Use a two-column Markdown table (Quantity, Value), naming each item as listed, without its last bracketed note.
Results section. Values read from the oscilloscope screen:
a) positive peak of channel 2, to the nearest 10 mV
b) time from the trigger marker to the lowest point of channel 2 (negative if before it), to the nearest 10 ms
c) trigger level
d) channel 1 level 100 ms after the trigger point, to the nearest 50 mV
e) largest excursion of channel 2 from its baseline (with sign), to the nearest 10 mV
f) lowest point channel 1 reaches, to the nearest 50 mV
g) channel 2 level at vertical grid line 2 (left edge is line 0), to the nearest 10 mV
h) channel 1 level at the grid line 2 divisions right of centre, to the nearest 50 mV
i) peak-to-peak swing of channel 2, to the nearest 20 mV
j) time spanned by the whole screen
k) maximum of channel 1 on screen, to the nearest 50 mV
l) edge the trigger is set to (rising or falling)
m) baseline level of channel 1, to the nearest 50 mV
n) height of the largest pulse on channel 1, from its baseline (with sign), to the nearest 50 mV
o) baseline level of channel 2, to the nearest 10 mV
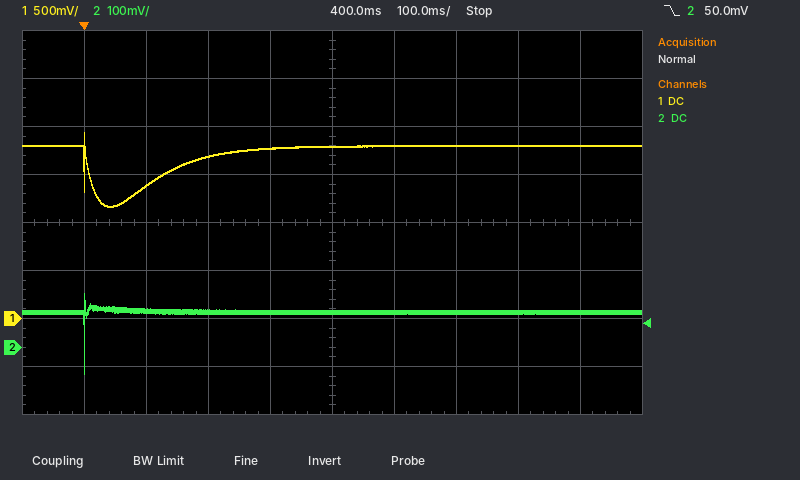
| Quantity | Value |
|---|---|
| positive peak of channel 2, to the nearest 10 mV | 110 mV |
| time from the trigger marker to the lowest point of channel 2 (negative if before it), to the nearest 10 ms | 0 ms |
| trigger level | 50.0 mV |
| channel 1 level 100 ms after the trigger point, to the nearest 50 mV | 1.40 V |
| largest excursion of channel 2 from its baseline (with sign), to the nearest 10 mV | -130 mV |
| lowest point channel 1 reaches, to the nearest 50 mV | 1.15 V |
| channel 2 level at vertical grid line 2 (left edge is line 0), to the nearest 10 mV | 80 mV |
| channel 1 level at the grid line 2 divisions right of centre, to the nearest 50 mV | 1.80 V |
| peak-to-peak swing of channel 2, to the nearest 20 mV | 160 mV |
| time spanned by the whole screen | 1 s |
| maximum of channel 1 on screen, to the nearest 50 mV | 1.95 V |
| edge the trigger is set to | falling |
| baseline level of channel 1, to the nearest 50 mV | 1.80 V |
| height of the largest pulse on channel 1, from its baseline (with sign), to the nearest 50 mV | -650 mV |
| baseline level of channel 2, to the nearest 10 mV | 70 mV |
